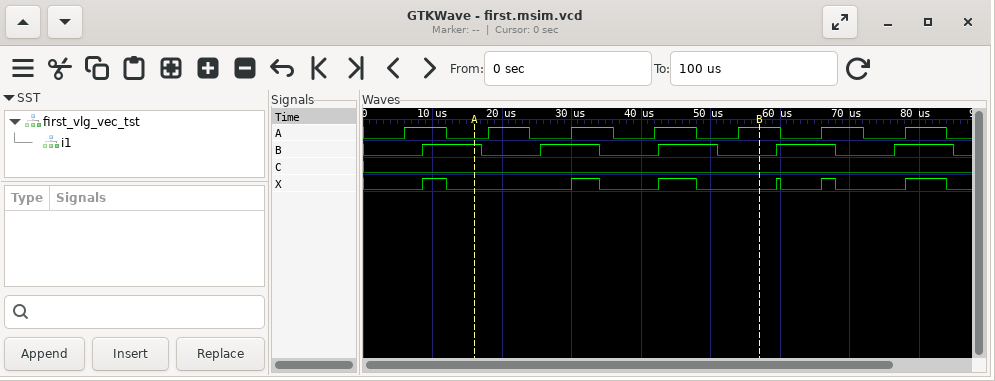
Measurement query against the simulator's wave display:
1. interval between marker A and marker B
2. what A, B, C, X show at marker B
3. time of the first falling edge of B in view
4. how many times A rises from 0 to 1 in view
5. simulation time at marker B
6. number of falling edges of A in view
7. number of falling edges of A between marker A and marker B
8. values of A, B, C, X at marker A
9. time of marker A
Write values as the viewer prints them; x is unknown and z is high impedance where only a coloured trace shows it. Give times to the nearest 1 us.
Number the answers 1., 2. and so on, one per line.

1. 41 us
2. A=1, B=0, C=0, X=0
3. 17 us
4. 7
5. 57 us
6. 7
7. 3
8. A=0, B=1, C=0, X=0
9. 16 us
